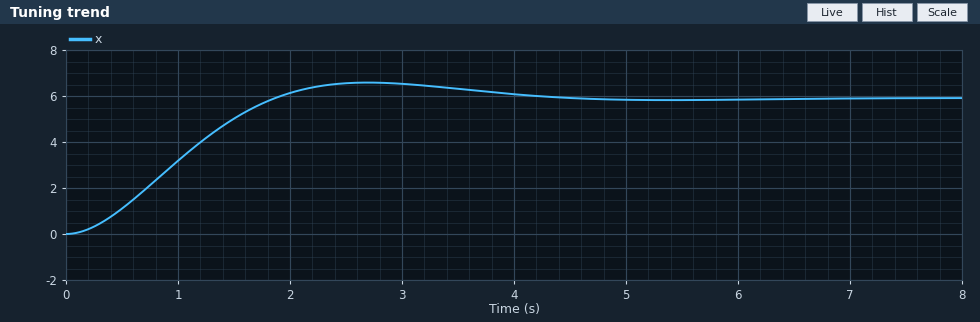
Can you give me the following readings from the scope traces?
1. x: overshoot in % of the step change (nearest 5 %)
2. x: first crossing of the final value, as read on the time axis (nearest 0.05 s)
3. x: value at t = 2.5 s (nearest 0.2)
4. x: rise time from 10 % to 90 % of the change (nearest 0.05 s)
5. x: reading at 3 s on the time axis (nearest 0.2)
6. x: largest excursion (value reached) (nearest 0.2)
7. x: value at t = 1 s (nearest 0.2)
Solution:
10 %
1.85 s
6.6
1.25 s
6.6
6.6
3.2
